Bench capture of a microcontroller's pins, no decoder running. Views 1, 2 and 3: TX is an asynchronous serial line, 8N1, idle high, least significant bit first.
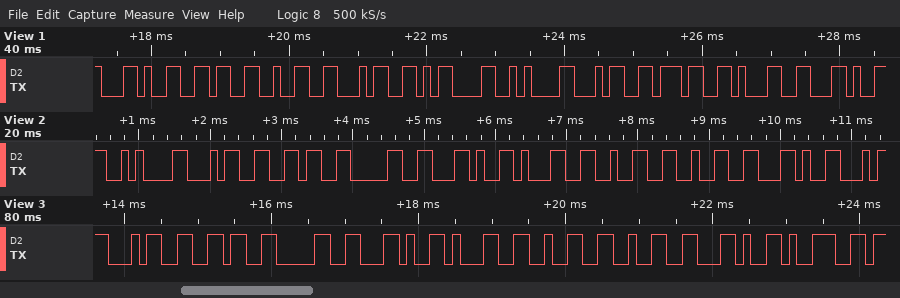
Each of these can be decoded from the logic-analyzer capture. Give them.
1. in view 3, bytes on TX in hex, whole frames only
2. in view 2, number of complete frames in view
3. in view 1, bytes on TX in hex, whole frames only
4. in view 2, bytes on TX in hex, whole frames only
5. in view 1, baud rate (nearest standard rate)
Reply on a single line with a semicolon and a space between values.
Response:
34 36 30 2C 31 32 32 2C 39; 9; 0x2C 0x36 0x32 0x34 0x0D 0x0A 0x34 0x37 0x31 0x2C; 0x0A 0x34 0x36 0x30 0x2C 0x31 0x32 0x32 0x2C; 9600 baud
